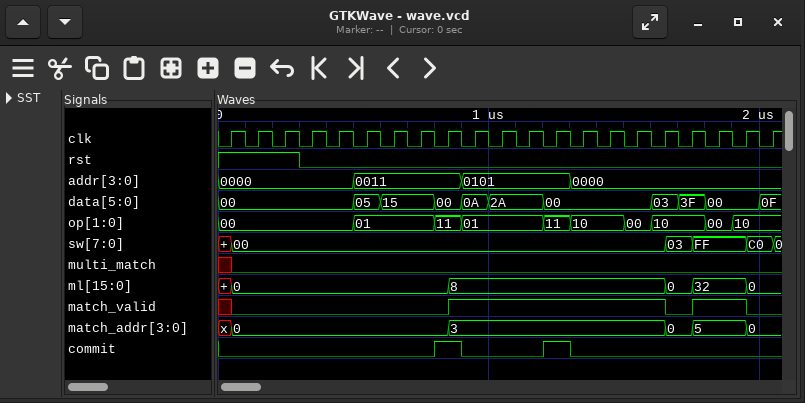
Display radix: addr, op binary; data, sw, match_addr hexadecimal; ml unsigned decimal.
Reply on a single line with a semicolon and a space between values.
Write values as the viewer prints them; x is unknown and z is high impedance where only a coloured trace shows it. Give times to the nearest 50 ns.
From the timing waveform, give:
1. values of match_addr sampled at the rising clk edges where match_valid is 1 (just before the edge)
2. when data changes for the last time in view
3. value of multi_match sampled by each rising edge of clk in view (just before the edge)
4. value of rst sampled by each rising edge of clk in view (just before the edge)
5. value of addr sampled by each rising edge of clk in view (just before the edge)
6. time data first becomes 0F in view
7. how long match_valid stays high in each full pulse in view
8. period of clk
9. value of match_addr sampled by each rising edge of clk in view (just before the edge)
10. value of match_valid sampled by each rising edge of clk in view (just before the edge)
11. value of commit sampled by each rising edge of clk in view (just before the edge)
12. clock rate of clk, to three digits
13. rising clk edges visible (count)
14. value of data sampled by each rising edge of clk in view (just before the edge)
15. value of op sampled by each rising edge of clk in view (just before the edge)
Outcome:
3, 3, 3, 3, 3, 3, 3, 3, 5, 5; 2000 ns; x 0 0 0 0 0 0 0 0 0 0 0 0 0 0 0 0 0 0 0 0; 1 1 1 0 0 0 0 0 0 0 0 0 0 0 0 0 0 0 0 0 0; 0000, 0000, 0000, 0000, 0000, 0011, 0011, 0011, 0011, 0101, 0101, 0101, 0101, 0000, 0000, 0000, 0000, 0000, 0000, 0000, 0000; 2000 ns; 800 ns, 200 ns; 100 ns; x, 0, 0, 0, 0, 0, 0, 0, 0, 3, 3, 3, 3, 3, 3, 3, 3, 0, 5, 5, 0; x 0 0 0 0 0 0 0 0 1 1 1 1 1 1 1 1 0 1 1 0; 0 0 0 0 0 0 0 0 1 0 0 0 1 0 0 0 0 0 0 0 0; 10.0 MHz; 21; 00, 00, 00, 00, 00, 05, 15, 15, 00, 0A, 2A, 2A, 00, 00, 00, 00, 03, 3F, 00, 00, 0F; 00, 00, 00, 00, 00, 01, 01, 01, 11, 01, 01, 01, 11, 10, 10, 00, 10, 10, 00, 10, 10
